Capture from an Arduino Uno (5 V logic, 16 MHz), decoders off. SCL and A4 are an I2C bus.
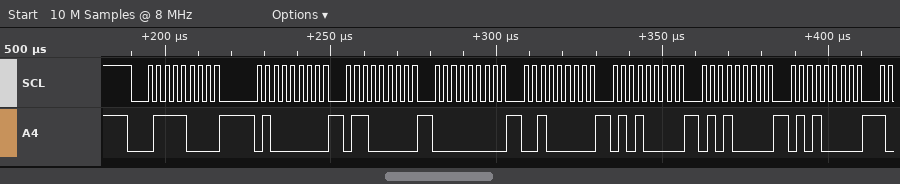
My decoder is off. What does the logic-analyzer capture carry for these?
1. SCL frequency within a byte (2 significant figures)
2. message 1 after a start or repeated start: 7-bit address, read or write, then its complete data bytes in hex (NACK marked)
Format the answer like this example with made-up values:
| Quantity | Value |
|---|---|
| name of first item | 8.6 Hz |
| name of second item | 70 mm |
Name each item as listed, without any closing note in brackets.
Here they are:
| Quantity | Value |
|---|---|
| SCL frequency within a byte | 400 kHz |
| message 1 after a start or repeated start: 7-bit address, read or write, then its complete data bytes in hex | 0x3C write: 40 60 00 20 50 50 50 |
